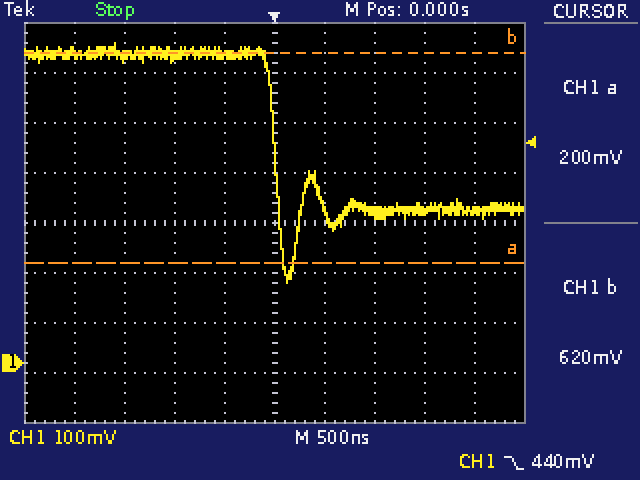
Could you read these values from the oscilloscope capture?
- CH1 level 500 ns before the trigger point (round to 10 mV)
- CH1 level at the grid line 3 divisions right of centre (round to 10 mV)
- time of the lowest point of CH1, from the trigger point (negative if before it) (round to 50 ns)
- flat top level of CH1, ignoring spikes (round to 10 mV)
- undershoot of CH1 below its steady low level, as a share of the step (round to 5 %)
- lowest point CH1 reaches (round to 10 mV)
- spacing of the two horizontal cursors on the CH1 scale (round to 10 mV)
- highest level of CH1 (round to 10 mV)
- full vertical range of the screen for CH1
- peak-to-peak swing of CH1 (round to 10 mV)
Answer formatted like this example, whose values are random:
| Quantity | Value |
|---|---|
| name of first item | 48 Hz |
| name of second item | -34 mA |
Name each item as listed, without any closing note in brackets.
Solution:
| Quantity | Value |
|---|---|
| CH1 level 500 ns before the trigger point | 620 mV |
| CH1 level at the grid line 3 divisions right of centre | 300 mV |
| time of the lowest point of CH1, from the trigger point (negative if before it) | +150 ns |
| flat top level of CH1, ignoring spikes | 620 mV |
| undershoot of CH1 below its steady low level, as a share of the step | 45 % |
| lowest point CH1 reaches | 160 mV |
| spacing of the two horizontal cursors on the CH1 scale | 420 mV |
| highest level of CH1 | 640 mV |
| full vertical range of the screen for CH1 | 800 mV |
| peak-to-peak swing of CH1 | 480 mV |
